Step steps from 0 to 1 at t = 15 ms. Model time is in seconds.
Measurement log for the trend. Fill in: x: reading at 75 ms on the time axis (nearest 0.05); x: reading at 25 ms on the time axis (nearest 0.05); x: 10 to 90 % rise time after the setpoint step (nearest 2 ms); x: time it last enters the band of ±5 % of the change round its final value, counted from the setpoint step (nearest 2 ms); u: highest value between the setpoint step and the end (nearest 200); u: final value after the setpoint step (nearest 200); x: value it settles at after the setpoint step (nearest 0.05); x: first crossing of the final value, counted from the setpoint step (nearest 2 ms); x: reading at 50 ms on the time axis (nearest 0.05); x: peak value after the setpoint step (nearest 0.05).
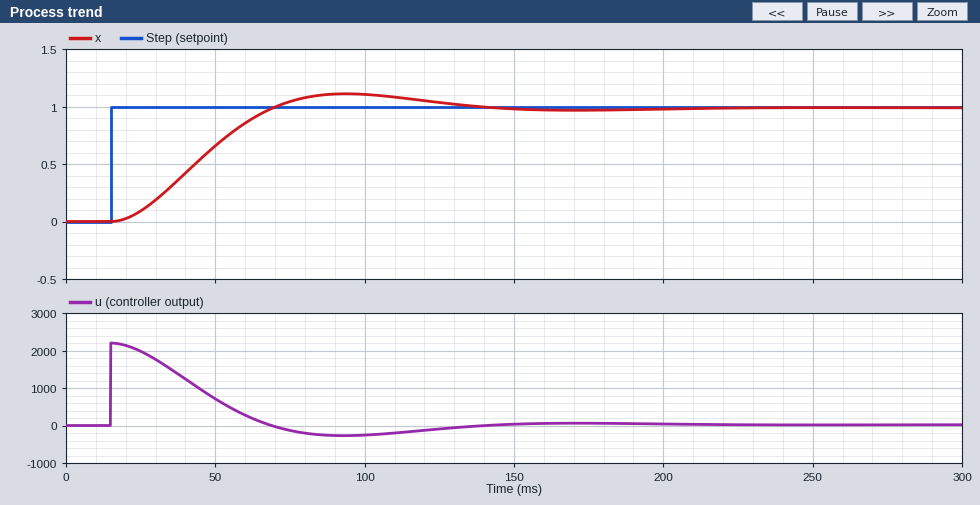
1.05
0.10
36 ms
108 ms
2200
0
1.00
54 ms
0.65
1.10
